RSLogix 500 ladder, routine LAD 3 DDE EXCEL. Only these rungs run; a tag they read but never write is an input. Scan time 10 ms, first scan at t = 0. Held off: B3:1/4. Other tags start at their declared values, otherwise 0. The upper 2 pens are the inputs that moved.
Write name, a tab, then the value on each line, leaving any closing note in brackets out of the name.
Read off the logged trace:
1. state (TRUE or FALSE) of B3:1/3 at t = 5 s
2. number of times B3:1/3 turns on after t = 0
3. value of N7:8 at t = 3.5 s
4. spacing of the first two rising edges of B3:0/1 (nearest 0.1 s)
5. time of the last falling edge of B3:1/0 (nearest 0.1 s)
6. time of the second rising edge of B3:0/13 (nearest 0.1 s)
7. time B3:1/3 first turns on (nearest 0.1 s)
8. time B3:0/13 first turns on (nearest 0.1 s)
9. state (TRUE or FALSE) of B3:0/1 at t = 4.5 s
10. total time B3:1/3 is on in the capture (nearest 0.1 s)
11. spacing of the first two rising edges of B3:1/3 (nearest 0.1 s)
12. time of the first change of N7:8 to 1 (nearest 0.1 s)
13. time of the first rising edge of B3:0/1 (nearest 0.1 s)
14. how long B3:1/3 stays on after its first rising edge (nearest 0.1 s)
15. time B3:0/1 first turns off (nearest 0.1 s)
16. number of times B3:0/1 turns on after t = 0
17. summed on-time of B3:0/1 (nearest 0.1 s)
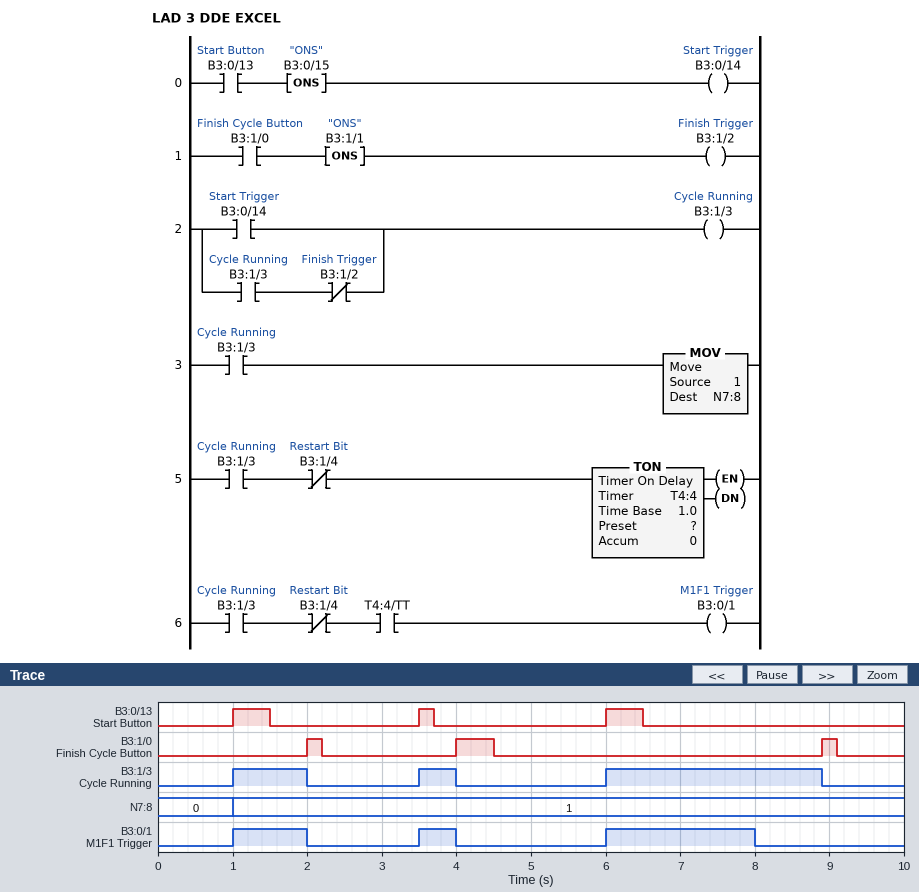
state (TRUE or FALSE) of B3:1/3 at t = 5 s	FALSE
number of times B3:1/3 turns on after t = 0	3
value of N7:8 at t = 3.5 s	1
spacing of the first two rising edges of B3:0/1	2.5 s
time of the last falling edge of B3:1/0	9.1 s
time of the second rising edge of B3:0/13	3.5 s
time B3:1/3 first turns on	1.0 s
time B3:0/13 first turns on	1.0 s
state (TRUE or FALSE) of B3:0/1 at t = 4.5 s	FALSE
total time B3:1/3 is on in the capture	4.4 s
spacing of the first two rising edges of B3:1/3	2.5 s
time of the first change of N7:8 to 1	1.0 s
time of the first rising edge of B3:0/1	1.0 s
how long B3:1/3 stays on after its first rising edge	1.0 s
time B3:0/1 first turns off	2.0 s
number of times B3:0/1 turns on after t = 0	3
summed on-time of B3:0/1	3.5 s
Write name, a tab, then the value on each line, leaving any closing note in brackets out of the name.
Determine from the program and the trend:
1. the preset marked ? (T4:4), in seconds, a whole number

the preset marked ? (T4:4), in seconds, a whole number	2 s
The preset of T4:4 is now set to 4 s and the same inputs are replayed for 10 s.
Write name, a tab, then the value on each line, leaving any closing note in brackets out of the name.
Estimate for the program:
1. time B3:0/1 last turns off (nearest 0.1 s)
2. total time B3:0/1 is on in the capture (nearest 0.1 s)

time B3:0/1 last turns off	8.9 s
total time B3:0/1 is on in the capture	4.4 s
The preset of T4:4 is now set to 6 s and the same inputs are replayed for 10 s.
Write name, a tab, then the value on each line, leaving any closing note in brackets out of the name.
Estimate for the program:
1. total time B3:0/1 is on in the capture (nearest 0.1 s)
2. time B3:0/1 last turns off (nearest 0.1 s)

total time B3:0/1 is on in the capture	4.4 s
time B3:0/1 last turns off	8.9 s
